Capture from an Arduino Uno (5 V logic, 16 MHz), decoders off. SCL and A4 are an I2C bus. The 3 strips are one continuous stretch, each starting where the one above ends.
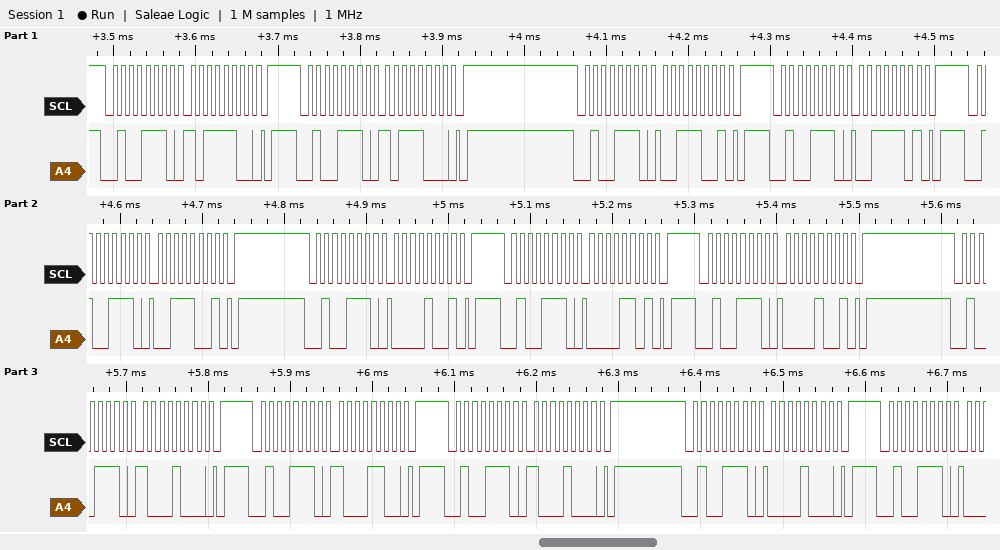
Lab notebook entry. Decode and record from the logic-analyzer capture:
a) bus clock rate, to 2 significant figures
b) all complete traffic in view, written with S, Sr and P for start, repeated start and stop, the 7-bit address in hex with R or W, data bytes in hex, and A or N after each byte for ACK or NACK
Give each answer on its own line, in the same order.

100 kHz
S 27W A BC A P S 27W A B8 A P S 27W A 39 A P S 27W A 3D A P S 27W A 39 A P S 27W A 09 A P S 27W A 0D A P S 27W A 09 A P S 27W A 88 A P S 27W A 8C A P S 27W A 88 A P S 27W A 08 A P S 27W A
